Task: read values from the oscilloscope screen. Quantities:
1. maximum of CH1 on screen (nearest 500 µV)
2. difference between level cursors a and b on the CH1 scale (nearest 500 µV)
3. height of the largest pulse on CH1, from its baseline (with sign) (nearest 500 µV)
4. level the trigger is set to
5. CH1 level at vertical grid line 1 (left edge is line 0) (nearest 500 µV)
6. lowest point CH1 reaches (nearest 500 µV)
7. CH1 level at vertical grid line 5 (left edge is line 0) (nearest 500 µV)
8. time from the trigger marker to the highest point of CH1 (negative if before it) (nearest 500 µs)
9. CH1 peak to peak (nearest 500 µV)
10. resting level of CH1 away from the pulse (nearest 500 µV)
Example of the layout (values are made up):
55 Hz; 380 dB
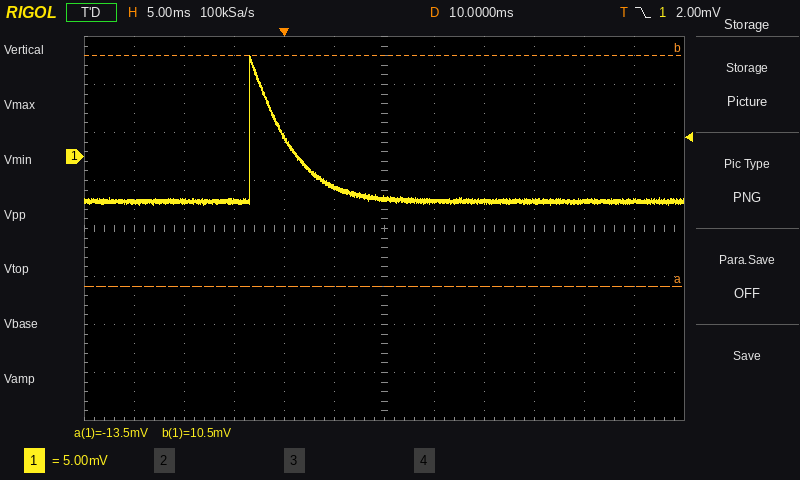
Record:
10.5 mV; 24.0 mV; +15.0 mV; 2.00 mV; -4.5 mV; -5.0 mV; -3.0 mV; -3.5 ms; 15.5 mV; -4.5 mV
